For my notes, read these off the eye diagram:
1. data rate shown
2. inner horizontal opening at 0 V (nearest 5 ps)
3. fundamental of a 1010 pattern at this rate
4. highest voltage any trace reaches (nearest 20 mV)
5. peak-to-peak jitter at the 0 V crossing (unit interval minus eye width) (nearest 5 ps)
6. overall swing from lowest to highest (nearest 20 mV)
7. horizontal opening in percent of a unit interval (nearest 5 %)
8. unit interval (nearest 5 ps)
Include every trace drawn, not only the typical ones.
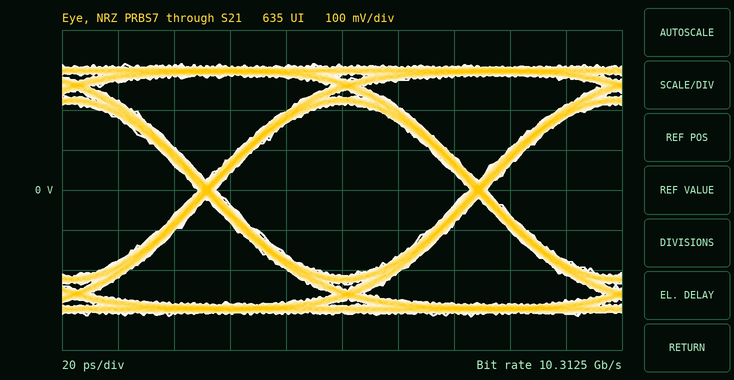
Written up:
10.3125 Gb/s
90 ps
5.15625 GHz
320 mV
5 ps
640 mV
95 %
95 ps
